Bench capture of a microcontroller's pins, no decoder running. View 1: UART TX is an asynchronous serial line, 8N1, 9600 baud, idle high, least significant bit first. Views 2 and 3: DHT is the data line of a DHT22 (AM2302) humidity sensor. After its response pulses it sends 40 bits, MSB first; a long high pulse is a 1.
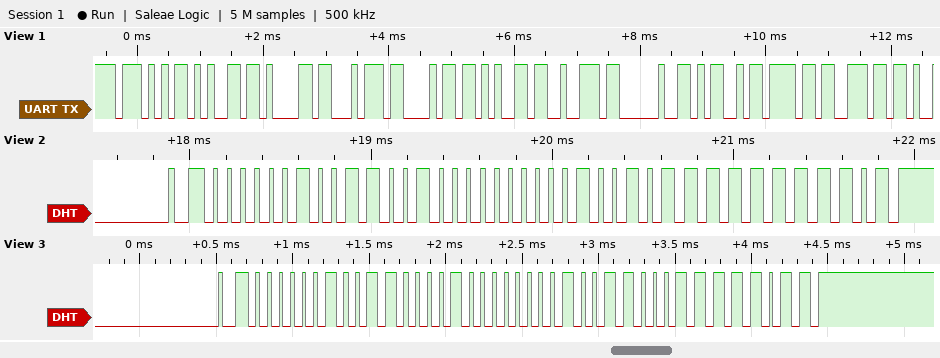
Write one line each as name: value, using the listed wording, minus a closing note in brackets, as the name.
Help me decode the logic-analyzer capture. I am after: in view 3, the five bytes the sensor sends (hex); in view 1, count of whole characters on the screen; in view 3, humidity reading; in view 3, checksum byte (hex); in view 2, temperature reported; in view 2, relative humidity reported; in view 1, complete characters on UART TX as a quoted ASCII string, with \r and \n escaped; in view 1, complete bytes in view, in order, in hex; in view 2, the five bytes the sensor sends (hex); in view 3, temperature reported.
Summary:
in view 3, the five bytes the sensor sends: 02 61 00 98 FB
in view 1, count of whole characters on the screen: 11
in view 3, humidity reading: 60.9 %
in view 3, checksum byte: 0xFB
in view 2, temperature reported: 15.1 °C
in view 2, relative humidity reported: 61.2 %
in view 1, complete characters on UART TX as a quoted ASCII string, with \r and \n escaped: "Weather Mon"
in view 1, complete bytes in view, in order, in hex: 57 65 61 74 68 65 72 20 4D 6F 6E
in view 2, the five bytes the sensor sends: 02 64 00 97 FD
in view 3, temperature reported: 15.2 °C
